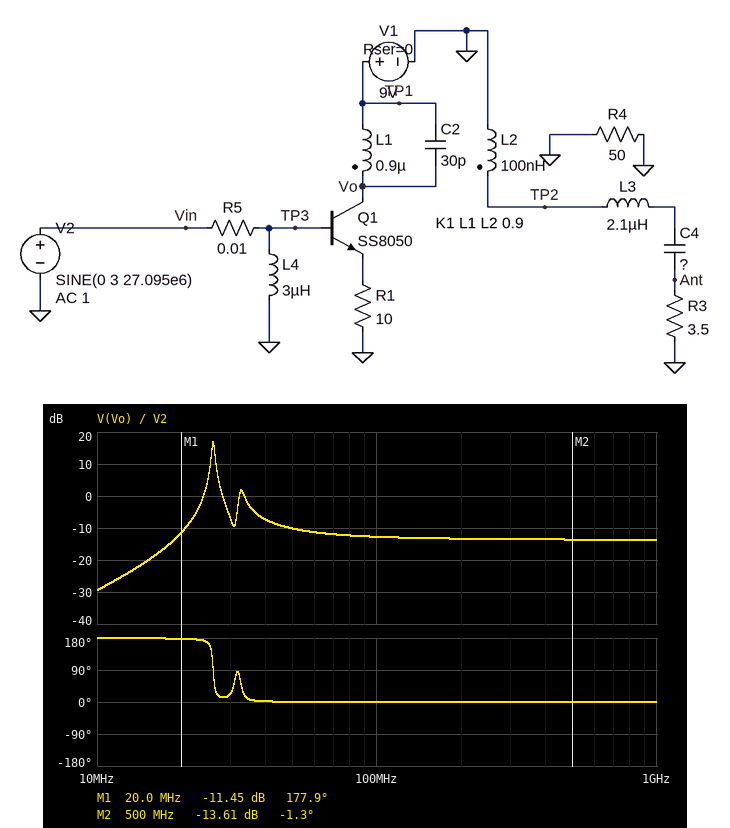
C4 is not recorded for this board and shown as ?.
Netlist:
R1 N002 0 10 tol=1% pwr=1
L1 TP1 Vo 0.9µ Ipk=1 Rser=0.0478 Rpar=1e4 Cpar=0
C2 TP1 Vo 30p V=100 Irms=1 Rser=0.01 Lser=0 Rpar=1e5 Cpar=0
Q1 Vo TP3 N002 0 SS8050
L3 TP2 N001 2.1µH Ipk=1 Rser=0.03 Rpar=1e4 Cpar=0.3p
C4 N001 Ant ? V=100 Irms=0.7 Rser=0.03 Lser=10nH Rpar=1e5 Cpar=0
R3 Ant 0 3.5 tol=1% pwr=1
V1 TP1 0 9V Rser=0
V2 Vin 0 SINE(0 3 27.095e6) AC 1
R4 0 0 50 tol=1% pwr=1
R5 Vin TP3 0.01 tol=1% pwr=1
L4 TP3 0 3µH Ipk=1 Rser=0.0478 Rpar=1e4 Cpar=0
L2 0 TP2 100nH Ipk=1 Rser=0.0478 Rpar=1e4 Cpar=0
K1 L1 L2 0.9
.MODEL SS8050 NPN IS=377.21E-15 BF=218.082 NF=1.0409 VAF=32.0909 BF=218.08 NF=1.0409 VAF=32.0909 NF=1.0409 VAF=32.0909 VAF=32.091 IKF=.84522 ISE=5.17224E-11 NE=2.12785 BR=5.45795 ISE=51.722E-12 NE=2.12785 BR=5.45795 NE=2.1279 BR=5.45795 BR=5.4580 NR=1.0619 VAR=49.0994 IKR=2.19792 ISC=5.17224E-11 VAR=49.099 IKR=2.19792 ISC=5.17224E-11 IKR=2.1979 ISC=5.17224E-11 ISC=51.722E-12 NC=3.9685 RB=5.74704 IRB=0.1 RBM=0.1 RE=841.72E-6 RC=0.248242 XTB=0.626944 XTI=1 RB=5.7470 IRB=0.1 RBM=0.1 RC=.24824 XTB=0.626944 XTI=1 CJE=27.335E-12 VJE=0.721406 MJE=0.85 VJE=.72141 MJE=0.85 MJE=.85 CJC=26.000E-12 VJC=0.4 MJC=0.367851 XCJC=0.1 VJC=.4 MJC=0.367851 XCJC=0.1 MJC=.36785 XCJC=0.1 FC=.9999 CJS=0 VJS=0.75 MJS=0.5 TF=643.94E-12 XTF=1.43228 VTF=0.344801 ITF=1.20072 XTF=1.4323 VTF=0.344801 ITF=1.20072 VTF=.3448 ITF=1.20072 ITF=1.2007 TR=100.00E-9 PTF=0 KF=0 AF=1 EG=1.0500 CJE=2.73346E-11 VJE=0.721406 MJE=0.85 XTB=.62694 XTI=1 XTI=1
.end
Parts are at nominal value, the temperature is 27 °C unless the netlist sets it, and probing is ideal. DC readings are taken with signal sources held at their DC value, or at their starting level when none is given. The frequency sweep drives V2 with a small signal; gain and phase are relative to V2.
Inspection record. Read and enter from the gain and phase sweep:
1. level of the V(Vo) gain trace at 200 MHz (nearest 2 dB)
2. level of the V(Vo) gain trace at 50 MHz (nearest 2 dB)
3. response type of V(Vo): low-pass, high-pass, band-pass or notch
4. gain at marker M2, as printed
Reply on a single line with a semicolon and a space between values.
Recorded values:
-14 dB; -10 dB; high-pass; -13.61 dB
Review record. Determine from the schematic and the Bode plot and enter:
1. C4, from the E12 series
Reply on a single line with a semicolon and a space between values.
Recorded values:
12 pF
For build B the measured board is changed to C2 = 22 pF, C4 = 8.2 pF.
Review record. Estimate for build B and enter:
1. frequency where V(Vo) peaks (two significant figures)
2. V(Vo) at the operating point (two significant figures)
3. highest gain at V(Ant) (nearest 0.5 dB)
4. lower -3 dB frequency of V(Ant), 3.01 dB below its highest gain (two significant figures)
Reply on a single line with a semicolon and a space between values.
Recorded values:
30 MHz; 9.0 V; -28.0 dB; 29 MHz
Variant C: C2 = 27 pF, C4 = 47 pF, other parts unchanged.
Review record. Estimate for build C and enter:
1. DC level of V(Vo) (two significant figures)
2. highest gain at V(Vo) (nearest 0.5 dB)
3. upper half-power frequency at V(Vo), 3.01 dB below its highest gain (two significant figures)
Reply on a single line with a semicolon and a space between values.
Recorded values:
9.0 V; 20.5 dB; 29 MHz
